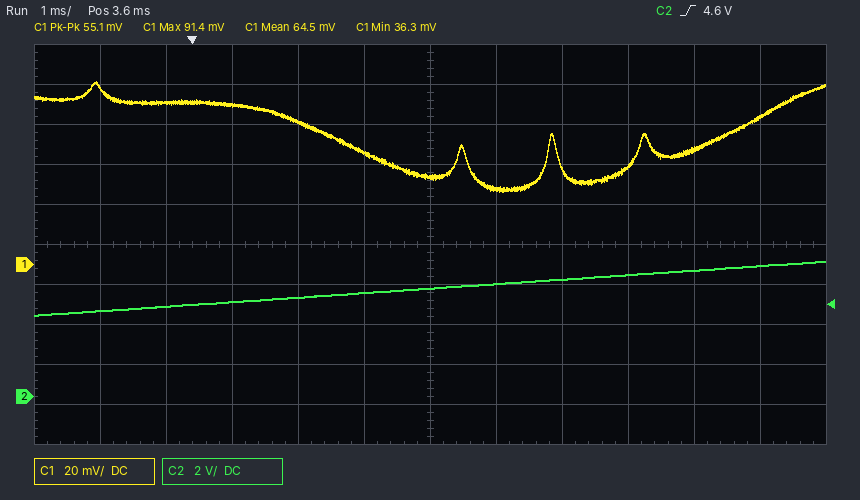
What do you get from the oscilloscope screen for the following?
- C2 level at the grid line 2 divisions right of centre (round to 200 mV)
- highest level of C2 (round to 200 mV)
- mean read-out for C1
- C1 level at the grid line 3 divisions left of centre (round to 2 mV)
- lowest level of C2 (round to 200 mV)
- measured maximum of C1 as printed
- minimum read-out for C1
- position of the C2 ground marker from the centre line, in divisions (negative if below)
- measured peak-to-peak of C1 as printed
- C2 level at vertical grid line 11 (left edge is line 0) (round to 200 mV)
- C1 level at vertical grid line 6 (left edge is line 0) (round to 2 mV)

5.8 V
6.8 V
64.5 mV
80 mV
4.0 V
91.4 mV
36.3 mV
-3.8 div
55.1 mV
6.6 V
44 mV
